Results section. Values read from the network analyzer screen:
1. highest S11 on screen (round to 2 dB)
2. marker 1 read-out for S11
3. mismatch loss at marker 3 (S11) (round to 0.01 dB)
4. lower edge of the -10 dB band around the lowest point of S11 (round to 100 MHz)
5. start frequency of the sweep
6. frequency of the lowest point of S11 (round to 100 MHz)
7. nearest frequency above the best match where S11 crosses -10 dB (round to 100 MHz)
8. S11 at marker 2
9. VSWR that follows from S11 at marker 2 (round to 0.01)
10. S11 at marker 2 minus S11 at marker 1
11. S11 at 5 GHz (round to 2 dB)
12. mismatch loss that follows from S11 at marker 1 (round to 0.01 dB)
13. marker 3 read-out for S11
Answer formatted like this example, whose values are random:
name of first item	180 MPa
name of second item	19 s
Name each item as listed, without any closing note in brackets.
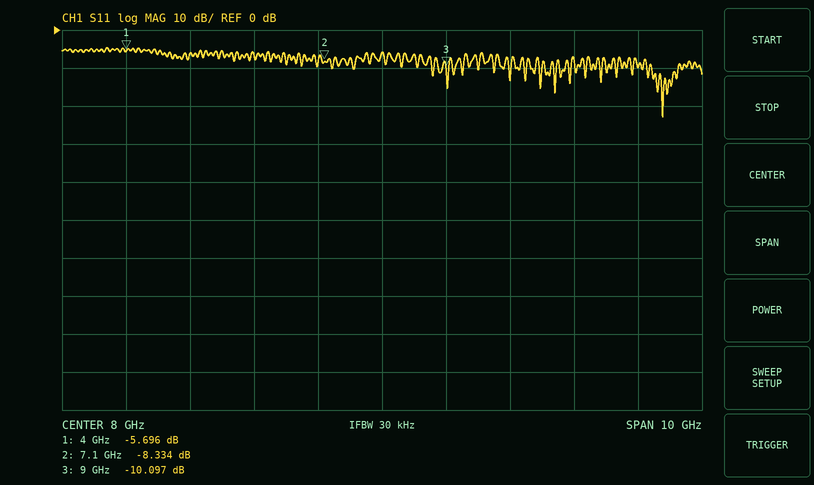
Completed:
highest S11 on screen	-4 dB
marker 1 read-out for S11	-5.696 dB
mismatch loss at marker 3 (S11)	0.45 dB
lower edge of the -10 dB band around the lowest point of S11	12.2 GHz
start frequency of the sweep	3 GHz
frequency of the lowest point of S11	12.4 GHz
nearest frequency above the best match where S11 crosses -10 dB	12.6 GHz
S11 at marker 2	-8.334 dB
VSWR that follows from S11 at marker 2	2.24
S11 at marker 2 minus S11 at marker 1	-2.638 dB
S11 at 5 GHz	-6 dB
mismatch loss that follows from S11 at marker 1	1.36 dB
marker 3 read-out for S11	-10.097 dB
